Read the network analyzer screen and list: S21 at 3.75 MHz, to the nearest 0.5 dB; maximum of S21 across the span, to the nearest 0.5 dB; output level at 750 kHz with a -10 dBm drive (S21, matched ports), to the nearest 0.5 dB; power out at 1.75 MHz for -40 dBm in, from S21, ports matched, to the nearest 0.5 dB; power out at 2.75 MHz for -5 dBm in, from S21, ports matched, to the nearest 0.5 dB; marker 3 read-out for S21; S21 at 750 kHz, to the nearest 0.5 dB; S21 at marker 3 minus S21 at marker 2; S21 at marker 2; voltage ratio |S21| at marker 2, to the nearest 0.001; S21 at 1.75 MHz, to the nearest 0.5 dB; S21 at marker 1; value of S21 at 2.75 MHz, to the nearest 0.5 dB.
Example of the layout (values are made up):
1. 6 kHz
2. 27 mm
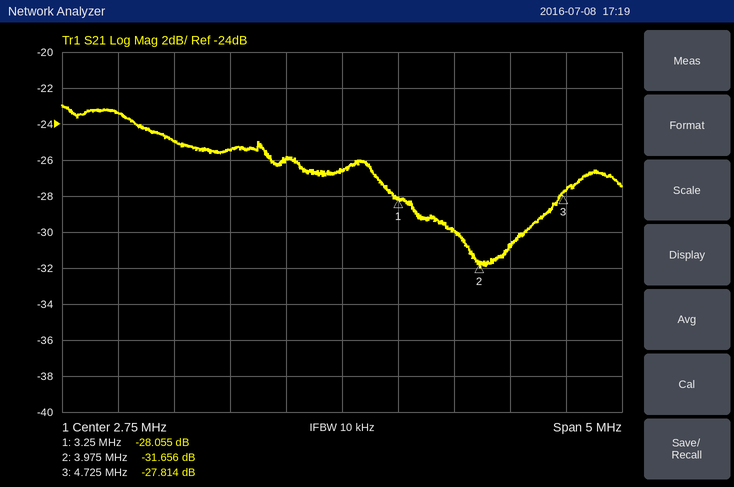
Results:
1. -30.0 dB
2. -23.0 dB
3. -33.5 dBm
4. -65.5 dBm
5. -31.5 dBm
6. -27.814 dB
7. -23.5 dB
8. 3.842 dB
9. -31.656 dB
10. 0.026
11. -25.5 dB
12. -28.055 dB
13. -26.5 dB
